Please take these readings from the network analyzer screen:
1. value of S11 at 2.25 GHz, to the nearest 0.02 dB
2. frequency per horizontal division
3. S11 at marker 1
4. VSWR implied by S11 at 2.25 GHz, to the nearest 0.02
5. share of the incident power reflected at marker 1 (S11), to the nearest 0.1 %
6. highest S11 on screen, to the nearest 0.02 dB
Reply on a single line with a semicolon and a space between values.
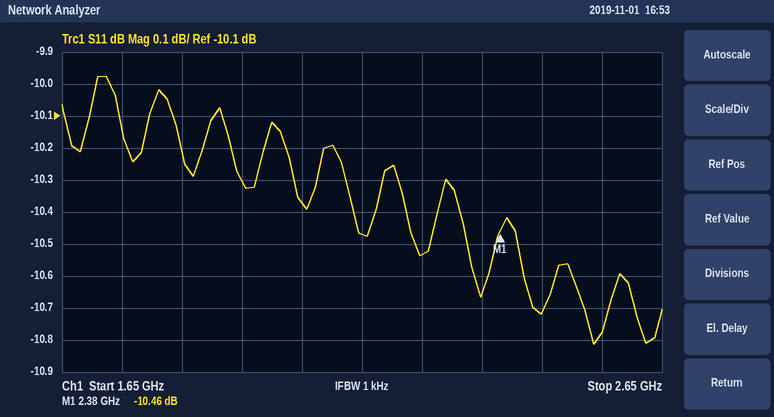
-10.54 dB; 100 MHz; -10.46 dB; 1.84; 9.0 %; -9.98 dB
